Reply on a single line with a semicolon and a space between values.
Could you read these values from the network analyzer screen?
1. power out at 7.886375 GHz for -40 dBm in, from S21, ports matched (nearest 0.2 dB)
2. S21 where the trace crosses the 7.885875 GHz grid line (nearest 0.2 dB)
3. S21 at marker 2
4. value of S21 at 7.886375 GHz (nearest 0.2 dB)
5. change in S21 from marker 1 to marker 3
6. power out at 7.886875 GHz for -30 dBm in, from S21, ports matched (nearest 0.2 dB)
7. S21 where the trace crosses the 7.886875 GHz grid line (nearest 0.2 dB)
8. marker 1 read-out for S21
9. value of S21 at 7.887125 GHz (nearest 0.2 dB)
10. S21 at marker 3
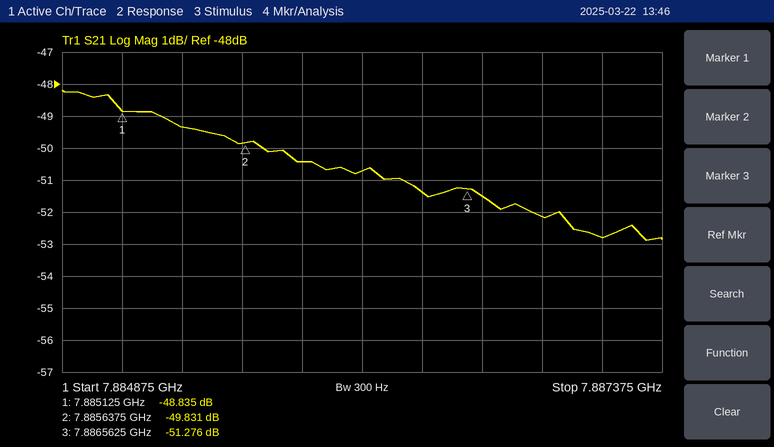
-91.4 dBm; -50.4 dB; -49.831 dB; -51.4 dB; -2.441 dB; -82.2 dBm; -52.2 dB; -48.835 dB; -52.8 dB; -51.276 dB
